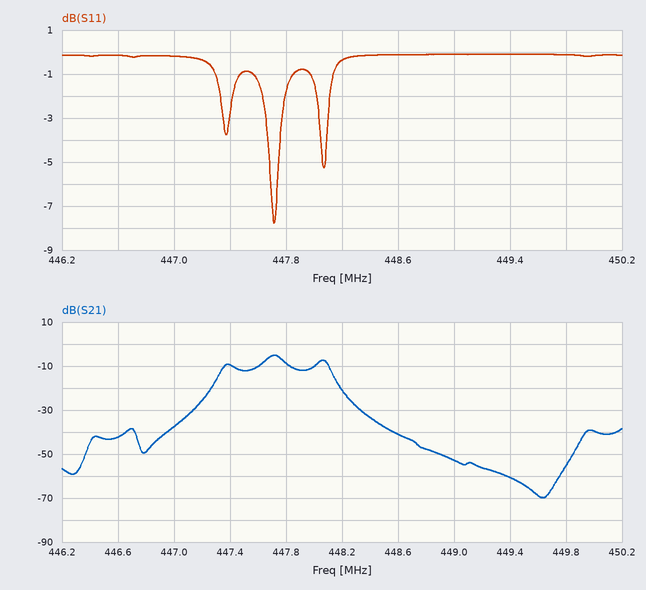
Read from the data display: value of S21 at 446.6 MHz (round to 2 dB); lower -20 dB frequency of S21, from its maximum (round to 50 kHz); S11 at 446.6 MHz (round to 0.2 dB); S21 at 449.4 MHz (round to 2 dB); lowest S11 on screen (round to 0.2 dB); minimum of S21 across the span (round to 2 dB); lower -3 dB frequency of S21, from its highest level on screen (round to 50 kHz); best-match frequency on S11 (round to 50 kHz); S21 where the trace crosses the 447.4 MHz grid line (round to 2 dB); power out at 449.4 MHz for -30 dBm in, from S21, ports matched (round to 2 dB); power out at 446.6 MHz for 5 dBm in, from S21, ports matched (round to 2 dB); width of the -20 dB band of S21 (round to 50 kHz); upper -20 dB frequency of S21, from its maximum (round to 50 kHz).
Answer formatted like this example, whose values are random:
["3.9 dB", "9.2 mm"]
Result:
["-42 dB", "447.20 MHz", "-0.2 dB", "-60 dB", "-7.8 dB", "-70 dB", "447.65 MHz", "447.70 MHz", "-10 dB", "-90 dBm", "-38 dBm", "1.05 MHz", "448.25 MHz"]
